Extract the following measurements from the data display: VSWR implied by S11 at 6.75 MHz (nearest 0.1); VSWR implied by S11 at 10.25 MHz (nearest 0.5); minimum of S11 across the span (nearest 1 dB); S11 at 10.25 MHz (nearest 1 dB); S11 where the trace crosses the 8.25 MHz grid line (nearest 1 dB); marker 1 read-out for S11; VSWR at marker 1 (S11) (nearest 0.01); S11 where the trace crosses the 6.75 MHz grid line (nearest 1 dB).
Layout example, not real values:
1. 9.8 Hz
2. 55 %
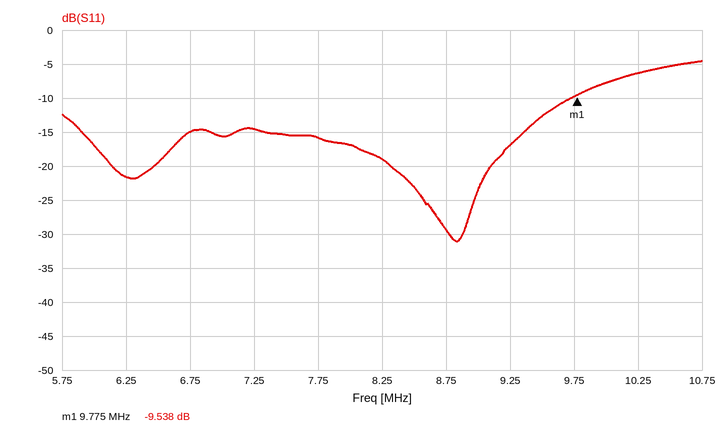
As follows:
1. 1.4
2. 3.0
3. -31 dB
4. -6 dB
5. -19 dB
6. -9.538 dB
7. 2.00
8. -15 dB
